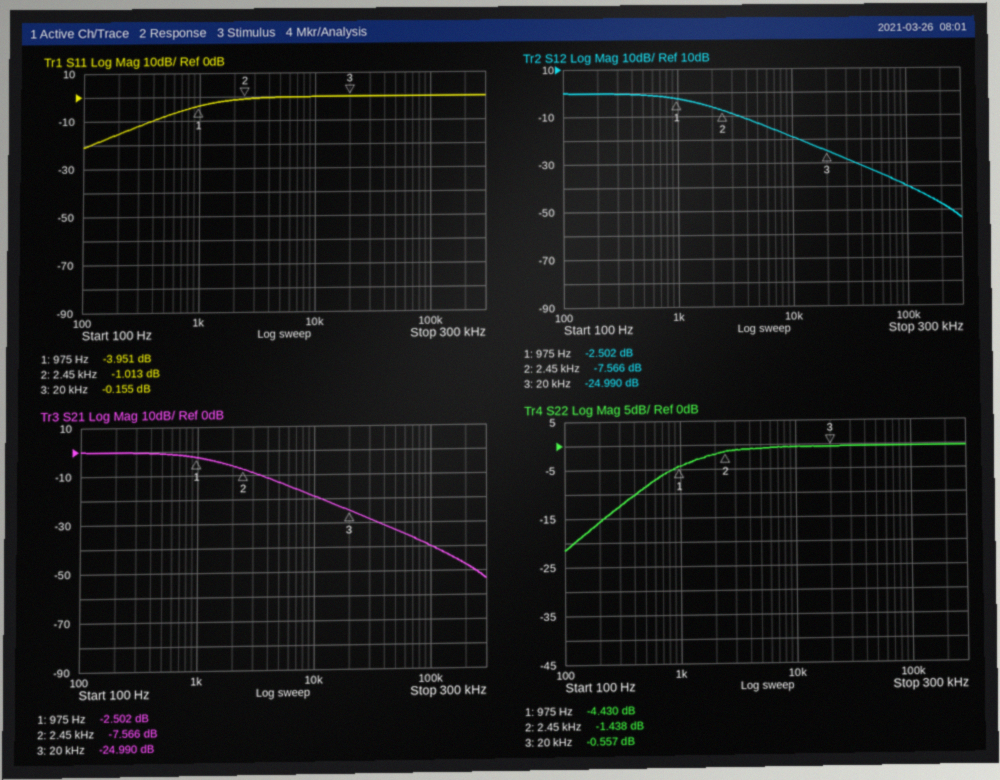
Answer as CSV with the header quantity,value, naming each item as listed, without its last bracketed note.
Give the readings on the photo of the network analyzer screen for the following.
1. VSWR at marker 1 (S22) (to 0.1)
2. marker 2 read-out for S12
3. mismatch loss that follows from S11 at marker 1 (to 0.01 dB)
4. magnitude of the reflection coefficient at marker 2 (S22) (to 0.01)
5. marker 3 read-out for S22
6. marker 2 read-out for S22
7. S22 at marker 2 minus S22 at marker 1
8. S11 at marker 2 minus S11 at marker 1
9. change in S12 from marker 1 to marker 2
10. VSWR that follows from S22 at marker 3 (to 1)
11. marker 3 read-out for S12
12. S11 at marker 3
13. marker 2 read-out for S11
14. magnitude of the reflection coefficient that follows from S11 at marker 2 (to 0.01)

quantity,value
VSWR at marker 1 (S22),4.0
marker 2 read-out for S12,-7.566 dB
mismatch loss that follows from S11 at marker 1,2.24 dB
magnitude of the reflection coefficient at marker 2 (S22),0.85
marker 3 read-out for S22,-0.557 dB
marker 2 read-out for S22,-1.438 dB
S22 at marker 2 minus S22 at marker 1,2.992 dB
S11 at marker 2 minus S11 at marker 1,2.938 dB
change in S12 from marker 1 to marker 2,-5.064 dB
VSWR that follows from S22 at marker 3,31
marker 3 read-out for S12,-24.990 dB
S11 at marker 3,-0.155 dB
marker 2 read-out for S11,-1.013 dB
magnitude of the reflection coefficient that follows from S11 at marker 2,0.89
